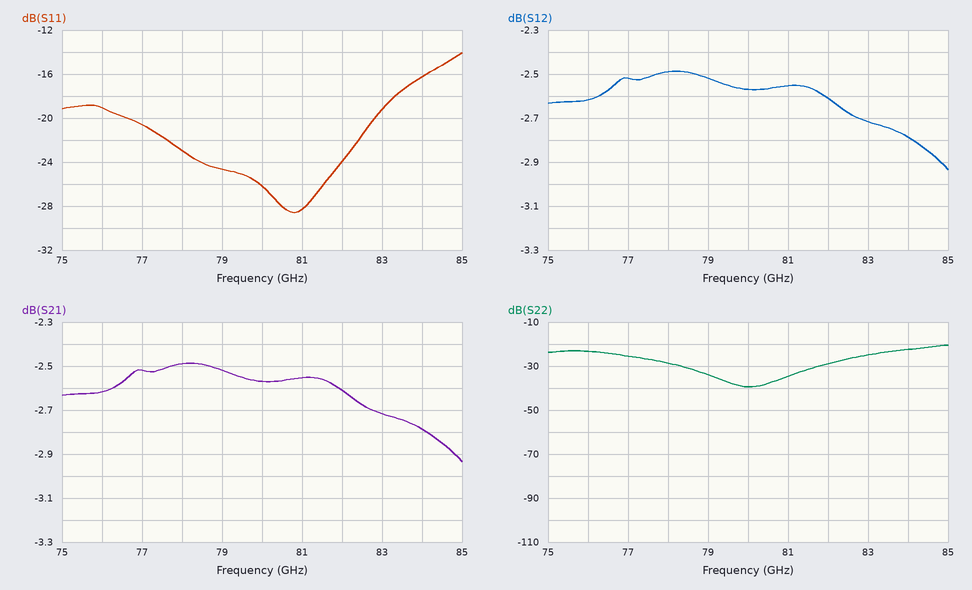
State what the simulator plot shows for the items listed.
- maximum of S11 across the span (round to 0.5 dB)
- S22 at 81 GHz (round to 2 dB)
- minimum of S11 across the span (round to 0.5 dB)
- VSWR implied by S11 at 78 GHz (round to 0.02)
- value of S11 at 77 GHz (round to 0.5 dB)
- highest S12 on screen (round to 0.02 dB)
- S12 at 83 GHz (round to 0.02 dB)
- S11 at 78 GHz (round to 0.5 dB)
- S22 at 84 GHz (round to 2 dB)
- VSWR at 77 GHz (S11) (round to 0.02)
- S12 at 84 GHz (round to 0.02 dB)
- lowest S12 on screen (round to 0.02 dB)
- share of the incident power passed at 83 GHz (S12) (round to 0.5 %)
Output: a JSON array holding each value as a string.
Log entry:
["-14.0 dB", "-34 dB", "-28.5 dB", "1.16", "-20.5 dB", "-2.48 dB", "-2.72 dB", "-23.0 dB", "-22 dB", "1.20", "-2.78 dB", "-2.94 dB", "53.5 %"]
